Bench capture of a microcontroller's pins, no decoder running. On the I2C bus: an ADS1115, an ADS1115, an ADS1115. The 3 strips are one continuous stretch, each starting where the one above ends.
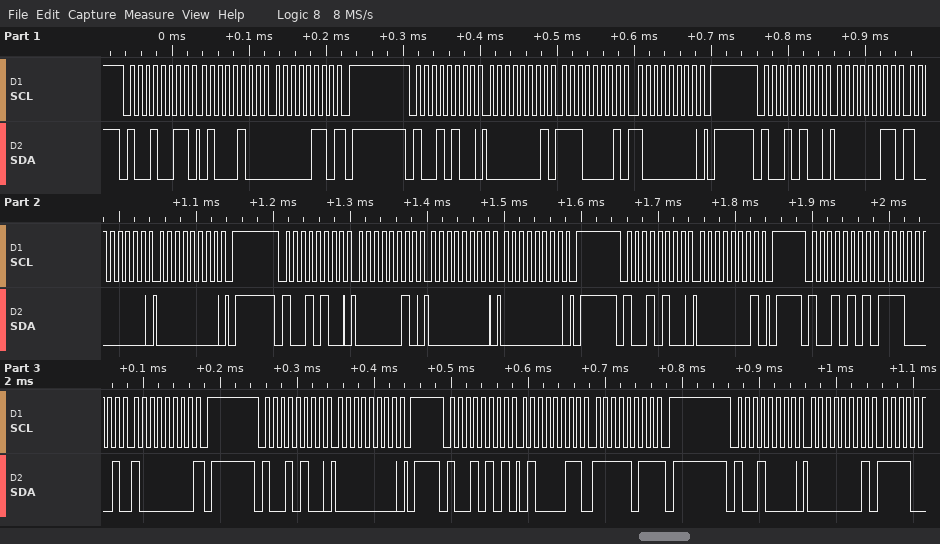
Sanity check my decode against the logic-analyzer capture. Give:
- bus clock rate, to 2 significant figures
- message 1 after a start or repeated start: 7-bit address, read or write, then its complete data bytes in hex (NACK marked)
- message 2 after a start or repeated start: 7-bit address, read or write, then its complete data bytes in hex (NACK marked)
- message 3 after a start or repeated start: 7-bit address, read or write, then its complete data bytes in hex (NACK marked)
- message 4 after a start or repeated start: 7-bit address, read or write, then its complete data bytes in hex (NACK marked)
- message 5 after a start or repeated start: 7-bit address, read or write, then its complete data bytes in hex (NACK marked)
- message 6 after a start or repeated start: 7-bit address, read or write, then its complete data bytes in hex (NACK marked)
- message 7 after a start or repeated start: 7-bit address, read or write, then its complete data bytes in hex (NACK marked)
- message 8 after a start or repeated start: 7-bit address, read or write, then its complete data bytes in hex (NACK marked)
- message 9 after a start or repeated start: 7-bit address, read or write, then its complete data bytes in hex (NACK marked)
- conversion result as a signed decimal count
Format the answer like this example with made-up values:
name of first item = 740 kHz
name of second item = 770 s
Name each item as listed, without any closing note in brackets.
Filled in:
bus clock rate, to 2 significant figures = 100 kHz
message 1 after a start or repeated start: 7-bit address, read or write, then its complete data bytes in hex = 0x49 read: 44 06 NACK
message 2 after a start or repeated start: 7-bit address, read or write, then its complete data bytes in hex = 0x4A write: 01 E1 80
message 3 after a start or repeated start: 7-bit address, read or write, then its complete data bytes in hex = 0x4A write: 03 80 00
message 4 after a start or repeated start: 7-bit address, read or write, then its complete data bytes in hex = 0x4A write: 02 00 00
message 5 after a start or repeated start: 7-bit address, read or write, then its complete data bytes in hex = 0x4A write: 01
message 6 after a start or repeated start: 7-bit address, read or write, then its complete data bytes in hex = 0x4A read: E1 80 NACK
message 7 after a start or repeated start: 7-bit address, read or write, then its complete data bytes in hex = 0x4A write: 00
message 8 after a start or repeated start: 7-bit address, read or write, then its complete data bytes in hex = 0x4A read: 43 FB NACK
message 9 after a start or repeated start: 7-bit address, read or write, then its complete data bytes in hex = 0x48 write: 01
conversion result as a signed decimal count = 17403
